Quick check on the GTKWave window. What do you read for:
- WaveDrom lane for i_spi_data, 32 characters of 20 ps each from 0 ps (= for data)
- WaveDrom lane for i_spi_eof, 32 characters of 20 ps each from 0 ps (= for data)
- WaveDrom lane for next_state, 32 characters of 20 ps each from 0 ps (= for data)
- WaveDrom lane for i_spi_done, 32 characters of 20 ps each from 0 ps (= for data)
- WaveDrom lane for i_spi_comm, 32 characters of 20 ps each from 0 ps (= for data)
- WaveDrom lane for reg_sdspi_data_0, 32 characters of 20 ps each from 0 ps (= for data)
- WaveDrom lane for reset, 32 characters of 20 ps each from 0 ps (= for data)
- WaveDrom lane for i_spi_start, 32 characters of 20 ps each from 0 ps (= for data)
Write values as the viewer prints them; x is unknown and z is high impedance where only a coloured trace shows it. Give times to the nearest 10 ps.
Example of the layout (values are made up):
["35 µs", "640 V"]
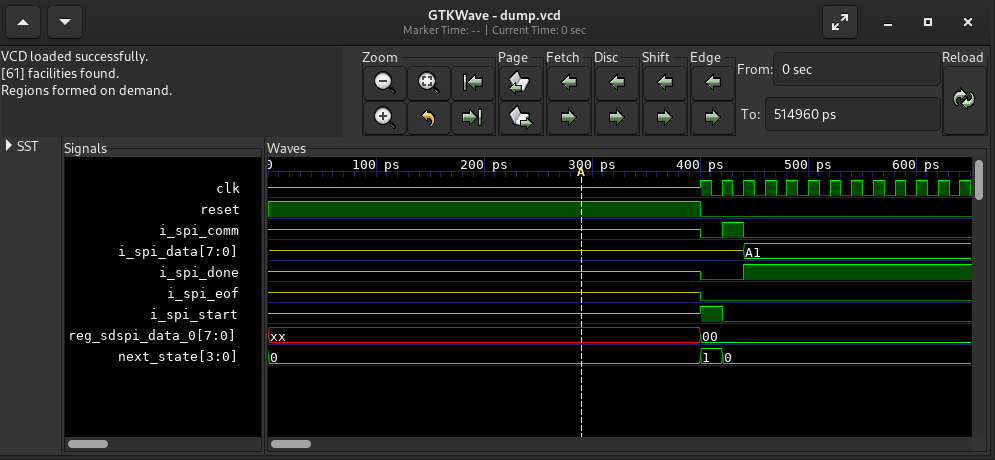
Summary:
["{name: 'i_spi_data', wave: 'z.....................=.........', data: 'A1'}", "{name: 'i_spi_eof', wave: 'z...................0...........'}", "{name: 'next_state', wave: '=...................==..........', data: '0 1 0'}", "{name: 'i_spi_done', wave: 'z...................0.1.........'}", "{name: 'i_spi_comm', wave: 'z...................010.........'}", "{name: 'reg_sdspi_data_0', wave: 'x...................=...........', data: '00'}", "{name: 'reset', wave: '1...................0...........'}", "{name: 'i_spi_start', wave: 'z...................10..........'}"]
